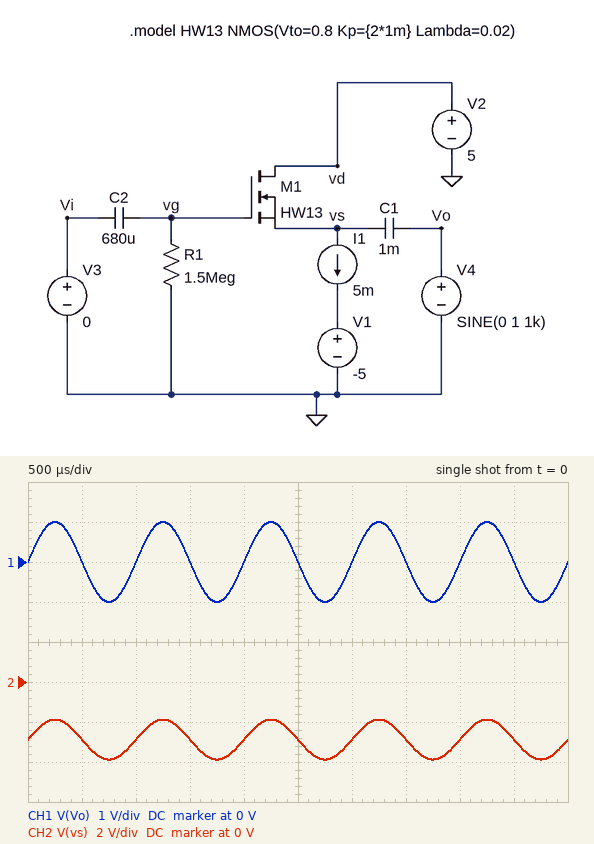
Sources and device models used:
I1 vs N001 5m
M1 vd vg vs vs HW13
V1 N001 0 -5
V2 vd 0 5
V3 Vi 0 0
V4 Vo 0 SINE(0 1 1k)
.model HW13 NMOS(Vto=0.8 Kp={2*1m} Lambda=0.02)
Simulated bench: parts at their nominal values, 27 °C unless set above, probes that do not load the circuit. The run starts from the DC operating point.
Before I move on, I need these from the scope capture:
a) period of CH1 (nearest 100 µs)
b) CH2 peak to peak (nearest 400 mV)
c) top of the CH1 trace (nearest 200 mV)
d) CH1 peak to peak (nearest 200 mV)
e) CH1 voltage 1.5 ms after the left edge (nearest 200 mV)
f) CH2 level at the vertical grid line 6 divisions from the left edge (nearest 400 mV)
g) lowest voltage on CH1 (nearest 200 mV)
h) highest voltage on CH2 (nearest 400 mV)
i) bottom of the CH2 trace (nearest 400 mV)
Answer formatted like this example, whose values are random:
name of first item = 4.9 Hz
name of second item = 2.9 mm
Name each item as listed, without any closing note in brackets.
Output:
period of CH1 = 1.0 ms
CH2 peak to peak = 2.0 V
top of the CH1 trace = 1.0 V
CH1 peak to peak = 2.0 V
CH1 voltage 1.5 ms after the left edge = 0 V
CH2 level at the vertical grid line 6 divisions from the left edge = -2.8 V
lowest voltage on CH1 = -1.0 V
highest voltage on CH2 = -2.0 V
bottom of the CH2 trace = -4.0 V
